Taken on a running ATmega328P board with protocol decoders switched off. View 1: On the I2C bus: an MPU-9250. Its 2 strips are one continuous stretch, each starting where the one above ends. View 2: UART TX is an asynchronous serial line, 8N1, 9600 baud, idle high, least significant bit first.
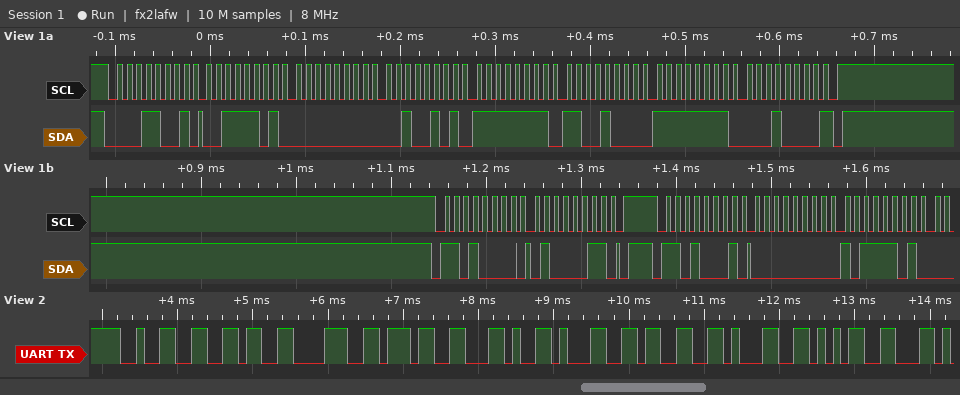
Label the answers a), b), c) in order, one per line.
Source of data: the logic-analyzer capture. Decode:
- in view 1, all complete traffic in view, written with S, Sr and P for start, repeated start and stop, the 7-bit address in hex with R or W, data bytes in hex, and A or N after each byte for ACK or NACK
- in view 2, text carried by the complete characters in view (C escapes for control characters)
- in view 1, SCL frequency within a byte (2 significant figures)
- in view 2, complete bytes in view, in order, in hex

a) S 0CR A 3D A 00 A 25 A FF A C8 A FF A 10 N P S 68W A 43 A P S 68R A 00 A BD A
b) "2687,1315"
c) 100 kHz
d) 0x32 0x36 0x38 0x37 0x2C 0x31 0x33 0x31 0x35
